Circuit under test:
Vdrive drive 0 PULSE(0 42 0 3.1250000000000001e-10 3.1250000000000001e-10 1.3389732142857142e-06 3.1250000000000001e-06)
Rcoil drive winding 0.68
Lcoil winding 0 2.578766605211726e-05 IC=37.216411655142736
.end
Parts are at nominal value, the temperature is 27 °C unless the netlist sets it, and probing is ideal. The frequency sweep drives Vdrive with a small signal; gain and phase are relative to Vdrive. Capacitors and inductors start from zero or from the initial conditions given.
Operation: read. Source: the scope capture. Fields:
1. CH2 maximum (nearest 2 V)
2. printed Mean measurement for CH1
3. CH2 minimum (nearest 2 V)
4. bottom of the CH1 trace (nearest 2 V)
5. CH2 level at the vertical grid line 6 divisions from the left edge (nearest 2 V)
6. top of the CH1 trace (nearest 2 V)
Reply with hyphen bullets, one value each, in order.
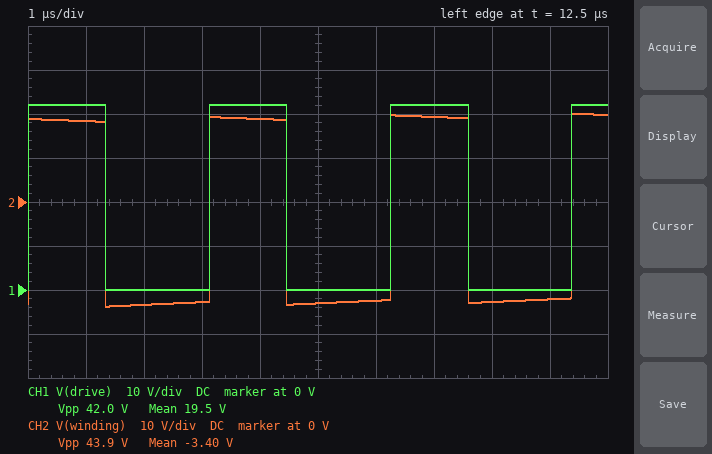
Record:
- 20 V
- 19.5 V
- -24 V
- 0 V
- -22 V
- 42 V
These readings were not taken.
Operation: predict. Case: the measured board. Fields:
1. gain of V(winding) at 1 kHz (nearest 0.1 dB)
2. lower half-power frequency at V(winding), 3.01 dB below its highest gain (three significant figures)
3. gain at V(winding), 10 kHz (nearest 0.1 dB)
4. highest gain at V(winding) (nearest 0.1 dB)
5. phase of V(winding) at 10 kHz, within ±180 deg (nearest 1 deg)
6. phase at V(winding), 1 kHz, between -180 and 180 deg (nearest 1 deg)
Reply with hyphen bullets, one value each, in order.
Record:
- -12.7 dB
- 4.20 kHz
- -0.7 dB
- 0 dB
- 23 deg
- 77 deg
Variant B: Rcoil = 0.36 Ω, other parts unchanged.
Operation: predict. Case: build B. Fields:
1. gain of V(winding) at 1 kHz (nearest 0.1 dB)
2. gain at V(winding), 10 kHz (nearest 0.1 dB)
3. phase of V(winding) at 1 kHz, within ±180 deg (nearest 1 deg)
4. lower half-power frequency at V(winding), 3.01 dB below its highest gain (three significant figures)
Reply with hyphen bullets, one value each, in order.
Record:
- -7.7 dB
- -0.2 dB
- 66 deg
- 2.22 kHz
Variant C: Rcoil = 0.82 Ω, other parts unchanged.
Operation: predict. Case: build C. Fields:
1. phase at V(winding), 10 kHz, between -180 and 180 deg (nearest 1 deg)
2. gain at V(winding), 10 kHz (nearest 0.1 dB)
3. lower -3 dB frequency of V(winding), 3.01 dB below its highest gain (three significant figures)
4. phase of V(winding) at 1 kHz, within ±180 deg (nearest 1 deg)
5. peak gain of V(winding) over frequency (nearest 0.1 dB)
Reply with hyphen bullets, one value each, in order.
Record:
- 27 deg
- -1.0 dB
- 5.06 kHz
- 79 deg
- 0 dB
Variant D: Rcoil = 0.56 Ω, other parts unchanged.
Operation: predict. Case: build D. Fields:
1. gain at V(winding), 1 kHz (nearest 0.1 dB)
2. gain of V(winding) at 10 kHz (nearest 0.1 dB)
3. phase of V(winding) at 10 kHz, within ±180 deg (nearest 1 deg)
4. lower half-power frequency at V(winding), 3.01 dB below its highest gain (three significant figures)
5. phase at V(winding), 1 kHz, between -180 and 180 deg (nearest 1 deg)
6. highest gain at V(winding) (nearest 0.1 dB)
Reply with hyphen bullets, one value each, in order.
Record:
- -11.1 dB
- -0.5 dB
- 19 deg
- 3.46 kHz
- 74 deg
- 0 dB
